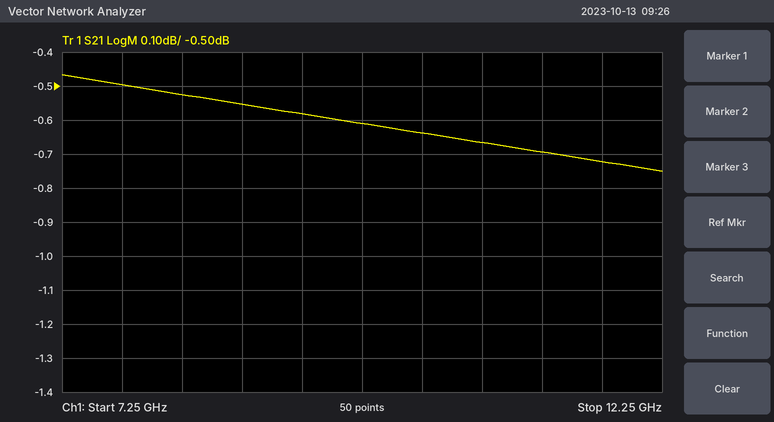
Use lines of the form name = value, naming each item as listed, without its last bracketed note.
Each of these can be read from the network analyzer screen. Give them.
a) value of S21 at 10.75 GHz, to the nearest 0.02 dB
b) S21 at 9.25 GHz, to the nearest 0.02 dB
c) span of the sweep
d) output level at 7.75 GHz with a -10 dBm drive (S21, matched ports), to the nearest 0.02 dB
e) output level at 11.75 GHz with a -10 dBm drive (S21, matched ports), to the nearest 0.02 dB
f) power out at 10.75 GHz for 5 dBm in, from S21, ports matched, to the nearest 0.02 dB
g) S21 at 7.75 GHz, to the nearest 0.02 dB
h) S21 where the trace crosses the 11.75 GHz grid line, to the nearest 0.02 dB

value of S21 at 10.75 GHz, to the nearest 0.02 dB = -0.66 dB
S21 at 9.25 GHz, to the nearest 0.02 dB = -0.58 dB
span of the sweep = 5 GHz
output level at 7.75 GHz with a -10 dBm drive (S21, matched ports), to the nearest 0.02 dB = -10.50 dBm
output level at 11.75 GHz with a -10 dBm drive (S21, matched ports), to the nearest 0.02 dB = -10.72 dBm
power out at 10.75 GHz for 5 dBm in, from S21, ports matched, to the nearest 0.02 dB = 4.34 dBm
S21 at 7.75 GHz, to the nearest 0.02 dB = -0.50 dB
S21 where the trace crosses the 11.75 GHz grid line, to the nearest 0.02 dB = -0.72 dB
